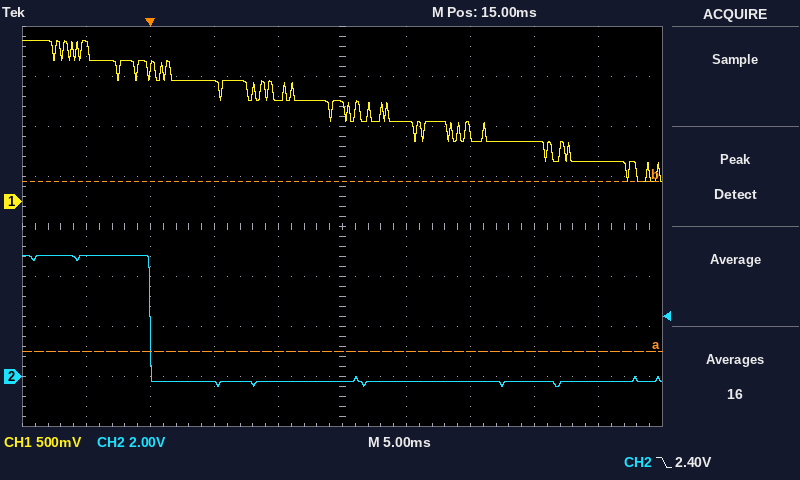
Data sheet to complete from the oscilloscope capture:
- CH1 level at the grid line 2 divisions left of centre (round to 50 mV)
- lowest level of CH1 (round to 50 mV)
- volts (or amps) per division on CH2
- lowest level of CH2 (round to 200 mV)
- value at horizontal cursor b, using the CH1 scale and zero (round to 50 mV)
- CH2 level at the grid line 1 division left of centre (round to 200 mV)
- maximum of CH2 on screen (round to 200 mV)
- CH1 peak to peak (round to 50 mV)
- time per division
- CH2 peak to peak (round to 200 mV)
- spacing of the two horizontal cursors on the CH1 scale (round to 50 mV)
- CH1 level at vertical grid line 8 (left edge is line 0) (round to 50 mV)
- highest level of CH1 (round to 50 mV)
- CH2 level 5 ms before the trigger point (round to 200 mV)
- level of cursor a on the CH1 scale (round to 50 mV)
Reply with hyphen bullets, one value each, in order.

- 1.20 V
- 200 mV
- 2 V
- -400 mV
- 200 mV
- -200 mV
- 4.8 V
- 1.40 V
- 5 ms
- 5.2 V
- 1.70 V
- 600 mV
- 1.60 V
- 4.8 V
- -1.50 V
